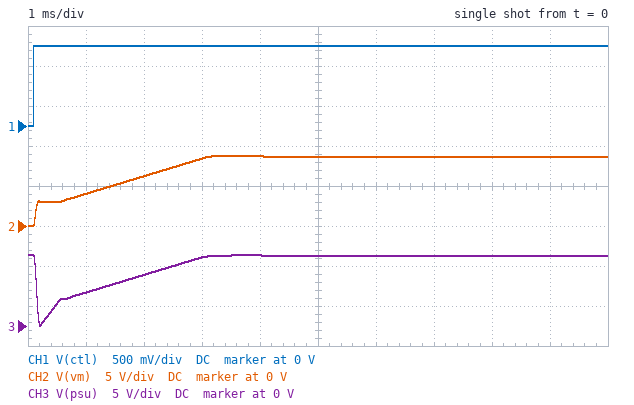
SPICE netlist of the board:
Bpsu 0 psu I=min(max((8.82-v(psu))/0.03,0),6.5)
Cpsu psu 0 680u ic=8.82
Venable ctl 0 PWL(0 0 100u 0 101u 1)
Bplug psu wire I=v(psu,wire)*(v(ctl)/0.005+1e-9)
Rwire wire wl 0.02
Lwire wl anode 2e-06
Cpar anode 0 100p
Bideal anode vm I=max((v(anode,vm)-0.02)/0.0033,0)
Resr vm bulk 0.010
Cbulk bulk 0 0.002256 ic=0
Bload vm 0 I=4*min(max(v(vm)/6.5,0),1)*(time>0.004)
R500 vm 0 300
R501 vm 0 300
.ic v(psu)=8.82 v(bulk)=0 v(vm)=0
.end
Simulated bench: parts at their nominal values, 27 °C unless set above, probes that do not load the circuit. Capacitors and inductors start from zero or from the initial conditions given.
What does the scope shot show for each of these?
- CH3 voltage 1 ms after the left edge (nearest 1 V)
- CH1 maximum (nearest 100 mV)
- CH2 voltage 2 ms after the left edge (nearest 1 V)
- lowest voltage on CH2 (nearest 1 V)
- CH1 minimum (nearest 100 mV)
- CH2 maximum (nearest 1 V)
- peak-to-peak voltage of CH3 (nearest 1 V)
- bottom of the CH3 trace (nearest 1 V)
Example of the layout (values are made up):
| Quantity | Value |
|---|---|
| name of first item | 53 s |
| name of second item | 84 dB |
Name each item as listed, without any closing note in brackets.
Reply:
| Quantity | Value |
|---|---|
| CH3 voltage 1 ms after the left edge | 4 V |
| CH1 maximum | 1.0 V |
| CH2 voltage 2 ms after the left edge | 6 V |
| lowest voltage on CH2 | 0 V |
| CH1 minimum | 0 V |
| CH2 maximum | 9 V |
| peak-to-peak voltage of CH3 | 9 V |
| bottom of the CH3 trace | 0 V |
